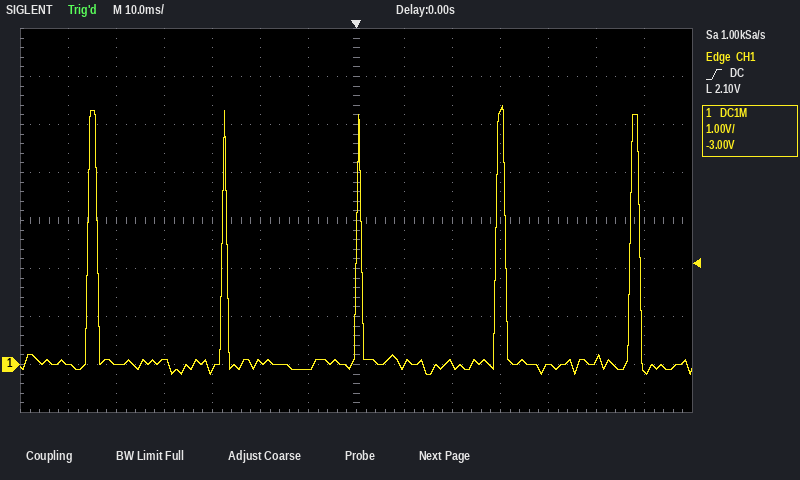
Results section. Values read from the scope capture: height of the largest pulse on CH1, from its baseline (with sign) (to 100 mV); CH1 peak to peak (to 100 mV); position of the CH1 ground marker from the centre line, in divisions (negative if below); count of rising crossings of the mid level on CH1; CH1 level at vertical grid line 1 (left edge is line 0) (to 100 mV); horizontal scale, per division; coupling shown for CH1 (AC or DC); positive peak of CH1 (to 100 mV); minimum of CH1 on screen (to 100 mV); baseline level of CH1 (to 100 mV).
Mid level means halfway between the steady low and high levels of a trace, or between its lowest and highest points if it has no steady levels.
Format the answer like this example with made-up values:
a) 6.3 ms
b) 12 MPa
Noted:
a) +5.4 V
b) 5.6 V
c) -3.0 div
d) 5
e) 0.0 V
f) 10 ms
g) DC
h) 5.4 V
i) -200 mV
j) 0.0 V
